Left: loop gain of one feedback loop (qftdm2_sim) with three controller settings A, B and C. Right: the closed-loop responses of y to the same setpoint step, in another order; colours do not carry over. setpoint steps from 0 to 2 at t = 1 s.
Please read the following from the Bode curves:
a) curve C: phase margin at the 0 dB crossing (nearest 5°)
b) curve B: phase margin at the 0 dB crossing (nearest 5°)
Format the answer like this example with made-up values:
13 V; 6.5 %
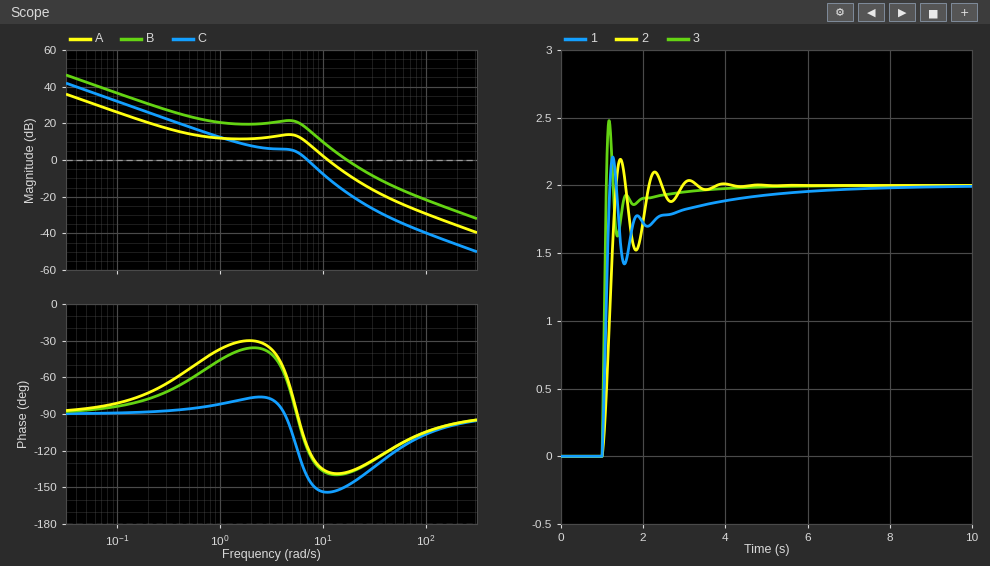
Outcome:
40°; 40°
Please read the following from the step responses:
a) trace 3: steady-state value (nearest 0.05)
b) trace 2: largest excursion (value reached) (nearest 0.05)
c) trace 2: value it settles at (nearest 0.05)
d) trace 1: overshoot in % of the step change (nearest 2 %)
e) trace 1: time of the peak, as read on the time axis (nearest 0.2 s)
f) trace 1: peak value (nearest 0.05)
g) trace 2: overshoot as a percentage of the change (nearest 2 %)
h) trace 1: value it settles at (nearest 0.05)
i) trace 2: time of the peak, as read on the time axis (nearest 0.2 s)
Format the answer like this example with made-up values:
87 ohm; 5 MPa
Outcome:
2.00; 2.20; 2.00; 10 %; 1.2 s; 2.20; 10 %; 2.00; 1.4 s
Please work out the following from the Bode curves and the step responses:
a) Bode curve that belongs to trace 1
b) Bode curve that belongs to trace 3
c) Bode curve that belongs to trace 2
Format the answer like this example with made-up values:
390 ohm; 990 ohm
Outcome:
A; B; C
